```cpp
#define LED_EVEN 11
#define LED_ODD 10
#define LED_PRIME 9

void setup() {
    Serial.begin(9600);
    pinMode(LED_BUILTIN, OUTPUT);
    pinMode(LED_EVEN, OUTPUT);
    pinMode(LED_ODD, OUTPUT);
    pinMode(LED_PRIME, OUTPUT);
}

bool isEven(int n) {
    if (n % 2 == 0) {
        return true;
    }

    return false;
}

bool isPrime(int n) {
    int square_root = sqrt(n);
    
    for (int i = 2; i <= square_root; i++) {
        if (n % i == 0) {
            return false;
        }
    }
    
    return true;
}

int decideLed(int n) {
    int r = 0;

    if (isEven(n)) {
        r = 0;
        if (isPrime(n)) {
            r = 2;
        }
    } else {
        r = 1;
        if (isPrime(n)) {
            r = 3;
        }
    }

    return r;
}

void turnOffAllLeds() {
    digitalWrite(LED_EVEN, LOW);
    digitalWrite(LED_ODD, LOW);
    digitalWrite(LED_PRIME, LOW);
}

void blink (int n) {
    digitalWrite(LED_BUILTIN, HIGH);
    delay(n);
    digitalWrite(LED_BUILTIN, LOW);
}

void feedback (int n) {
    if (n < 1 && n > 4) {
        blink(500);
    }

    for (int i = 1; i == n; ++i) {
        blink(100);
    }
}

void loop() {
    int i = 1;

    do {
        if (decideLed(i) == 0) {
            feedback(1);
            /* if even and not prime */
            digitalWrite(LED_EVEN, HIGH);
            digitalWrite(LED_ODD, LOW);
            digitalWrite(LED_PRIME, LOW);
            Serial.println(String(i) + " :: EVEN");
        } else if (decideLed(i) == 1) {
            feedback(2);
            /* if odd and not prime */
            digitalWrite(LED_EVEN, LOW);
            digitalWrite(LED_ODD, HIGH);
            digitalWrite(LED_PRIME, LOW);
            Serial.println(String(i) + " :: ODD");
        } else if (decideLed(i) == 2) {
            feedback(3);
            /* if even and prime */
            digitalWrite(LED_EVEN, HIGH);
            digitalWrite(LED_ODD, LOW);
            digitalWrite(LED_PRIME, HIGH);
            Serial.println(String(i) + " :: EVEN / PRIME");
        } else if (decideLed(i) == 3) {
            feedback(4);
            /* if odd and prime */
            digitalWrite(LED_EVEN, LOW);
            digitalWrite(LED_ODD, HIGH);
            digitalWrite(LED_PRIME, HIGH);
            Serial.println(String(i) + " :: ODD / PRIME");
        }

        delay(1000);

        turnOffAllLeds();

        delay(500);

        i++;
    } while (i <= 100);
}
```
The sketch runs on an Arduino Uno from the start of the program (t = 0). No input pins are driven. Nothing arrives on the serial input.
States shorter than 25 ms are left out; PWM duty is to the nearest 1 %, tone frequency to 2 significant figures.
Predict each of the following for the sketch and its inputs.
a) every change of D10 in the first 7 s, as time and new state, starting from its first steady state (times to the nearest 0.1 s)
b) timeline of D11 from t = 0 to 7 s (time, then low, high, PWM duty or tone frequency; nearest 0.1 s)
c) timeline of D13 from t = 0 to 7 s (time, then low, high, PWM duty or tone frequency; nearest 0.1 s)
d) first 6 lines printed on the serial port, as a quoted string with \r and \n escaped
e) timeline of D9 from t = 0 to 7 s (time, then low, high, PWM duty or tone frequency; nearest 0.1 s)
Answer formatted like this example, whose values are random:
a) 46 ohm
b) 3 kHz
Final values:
a) 0 s high; 1 s low; 3 s high; 4 s low; 6.1 s high
b) 0 s low; 1.5 s high; 2.5 s low; 4.6 s high; 5.6 s low
c) 0 s low; 4.5 s high; 4.6 s low
d) "1 :: ODD / PRIME\r\n2 :: EVEN / PRIME\r\n3 :: ODD / PRIME\r\n4 :: EVEN\r\n5 :: ODD / PRIME\r\n6 :: EVEN\r\n"
e) 0 s high; 1 s low; 1.5 s high; 2.5 s low; 3 s high; 4 s low; 6.1 s high
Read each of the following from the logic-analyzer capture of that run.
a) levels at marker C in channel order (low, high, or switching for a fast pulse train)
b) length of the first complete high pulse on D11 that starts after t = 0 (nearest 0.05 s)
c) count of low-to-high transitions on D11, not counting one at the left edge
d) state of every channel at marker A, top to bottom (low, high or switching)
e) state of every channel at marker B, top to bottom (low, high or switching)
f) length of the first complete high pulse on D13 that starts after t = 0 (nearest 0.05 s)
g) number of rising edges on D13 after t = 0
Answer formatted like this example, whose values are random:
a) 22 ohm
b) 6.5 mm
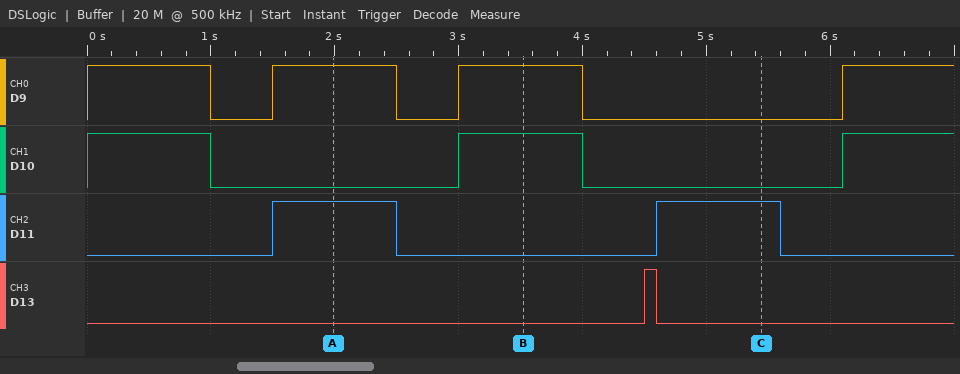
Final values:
a) D9 low, D10 low, D11 high, D13 low
b) 1.00 s
c) 2
d) D9 high, D10 low, D11 high, D13 low
e) D9 high, D10 high, D11 low, D13 low
f) 0.10 s
g) 1
